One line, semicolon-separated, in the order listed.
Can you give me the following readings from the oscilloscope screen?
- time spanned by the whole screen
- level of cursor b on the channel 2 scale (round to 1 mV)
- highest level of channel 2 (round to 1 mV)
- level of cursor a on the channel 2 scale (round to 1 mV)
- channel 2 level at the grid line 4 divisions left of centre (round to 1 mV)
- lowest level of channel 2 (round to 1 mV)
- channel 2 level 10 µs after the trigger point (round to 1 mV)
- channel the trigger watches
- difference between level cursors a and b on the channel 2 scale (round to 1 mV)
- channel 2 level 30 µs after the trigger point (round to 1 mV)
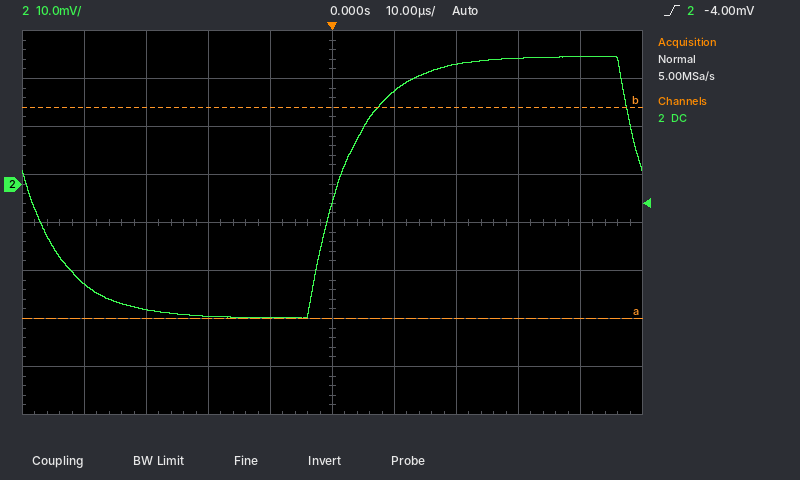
100 µs; 16 mV; 27 mV; -28 mV; -21 mV; -28 mV; 19 mV; channel 2; 44 mV; 26 mV
